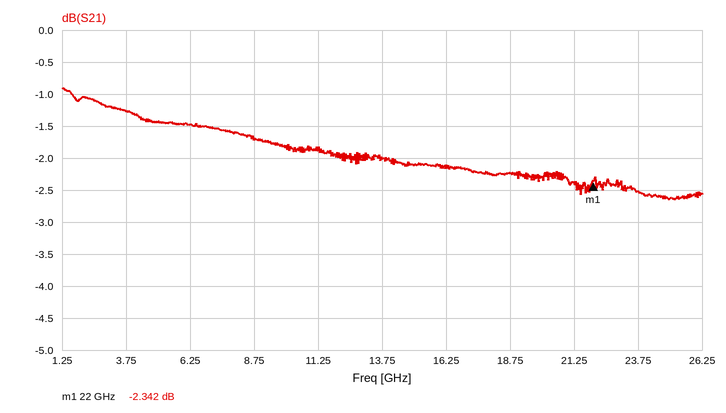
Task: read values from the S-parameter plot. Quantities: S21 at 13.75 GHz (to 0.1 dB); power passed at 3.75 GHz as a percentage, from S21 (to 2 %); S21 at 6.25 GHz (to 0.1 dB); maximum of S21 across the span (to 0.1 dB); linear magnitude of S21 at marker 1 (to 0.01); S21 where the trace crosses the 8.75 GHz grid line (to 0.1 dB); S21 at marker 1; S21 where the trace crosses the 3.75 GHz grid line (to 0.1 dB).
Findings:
-2.0 dB
74 %
-1.5 dB
-0.9 dB
0.76
-1.7 dB
-2.342 dB
-1.3 dB
